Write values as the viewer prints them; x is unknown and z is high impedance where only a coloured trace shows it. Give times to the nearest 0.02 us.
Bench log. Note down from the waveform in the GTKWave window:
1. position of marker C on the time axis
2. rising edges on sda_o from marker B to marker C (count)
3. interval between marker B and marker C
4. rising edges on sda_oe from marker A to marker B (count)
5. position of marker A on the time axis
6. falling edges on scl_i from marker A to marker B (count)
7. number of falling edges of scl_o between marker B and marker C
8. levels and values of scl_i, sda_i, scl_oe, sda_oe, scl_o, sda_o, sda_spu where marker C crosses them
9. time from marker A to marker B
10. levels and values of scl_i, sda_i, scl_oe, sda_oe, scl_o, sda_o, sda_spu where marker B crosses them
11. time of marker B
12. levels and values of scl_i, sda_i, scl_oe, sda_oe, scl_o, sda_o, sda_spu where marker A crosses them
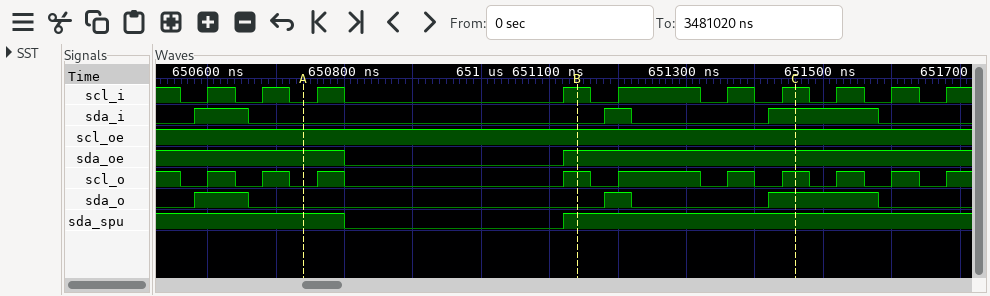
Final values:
651.46 us
2
0.32 us
1
650.74 us
1
3
scl_i=1, sda_i=1, scl_oe=1, sda_oe=1, scl_o=1, sda_o=1, sda_spu=1
0.4 us
scl_i=1, sda_i=0, scl_oe=1, sda_oe=1, scl_o=1, sda_o=0, sda_spu=1
651.14 us
scl_i=0, sda_i=0, scl_oe=1, sda_oe=1, scl_o=0, sda_o=0, sda_spu=1
